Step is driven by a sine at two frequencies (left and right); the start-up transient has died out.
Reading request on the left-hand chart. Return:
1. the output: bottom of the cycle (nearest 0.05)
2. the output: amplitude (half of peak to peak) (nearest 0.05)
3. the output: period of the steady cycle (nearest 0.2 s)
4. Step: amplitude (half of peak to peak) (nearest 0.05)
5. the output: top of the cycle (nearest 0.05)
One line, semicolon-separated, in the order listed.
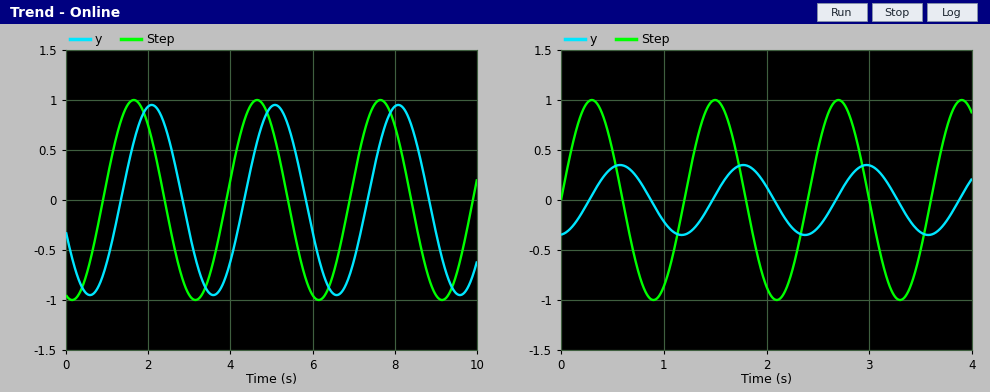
-0.95; 0.95; 3.0 s; 1.00; 0.95
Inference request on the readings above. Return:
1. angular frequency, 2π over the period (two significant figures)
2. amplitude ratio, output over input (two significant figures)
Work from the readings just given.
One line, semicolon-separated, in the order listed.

2.1 rad/s; 0.95
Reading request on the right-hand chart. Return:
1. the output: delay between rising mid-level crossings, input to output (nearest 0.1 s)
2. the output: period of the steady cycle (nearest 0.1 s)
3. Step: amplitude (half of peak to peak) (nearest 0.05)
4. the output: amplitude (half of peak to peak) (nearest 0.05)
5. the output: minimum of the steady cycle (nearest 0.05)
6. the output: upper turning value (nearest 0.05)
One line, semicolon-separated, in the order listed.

0.3 s; 1.2 s; 1.00; 0.35; -0.35; 0.35
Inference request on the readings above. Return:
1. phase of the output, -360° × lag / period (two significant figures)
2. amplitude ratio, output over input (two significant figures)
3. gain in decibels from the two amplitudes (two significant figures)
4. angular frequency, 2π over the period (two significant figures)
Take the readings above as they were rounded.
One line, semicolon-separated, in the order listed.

-90°; 0.35; -9.1 dB; 5.2 rad/s
